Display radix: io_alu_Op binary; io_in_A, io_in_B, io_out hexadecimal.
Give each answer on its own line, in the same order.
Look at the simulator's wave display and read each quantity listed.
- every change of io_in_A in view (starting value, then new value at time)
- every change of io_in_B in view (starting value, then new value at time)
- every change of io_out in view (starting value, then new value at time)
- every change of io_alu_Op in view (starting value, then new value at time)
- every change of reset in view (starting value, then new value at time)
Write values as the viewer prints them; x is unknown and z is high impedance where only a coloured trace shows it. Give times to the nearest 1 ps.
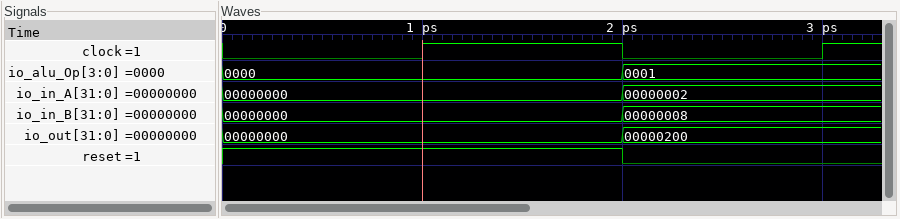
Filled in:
00000000, 00000002 at 2 ps
00000000, 00000008 at 2 ps
00000000, 00000200 at 2 ps
0000, 0001 at 2 ps
1, 0 at 2 ps
